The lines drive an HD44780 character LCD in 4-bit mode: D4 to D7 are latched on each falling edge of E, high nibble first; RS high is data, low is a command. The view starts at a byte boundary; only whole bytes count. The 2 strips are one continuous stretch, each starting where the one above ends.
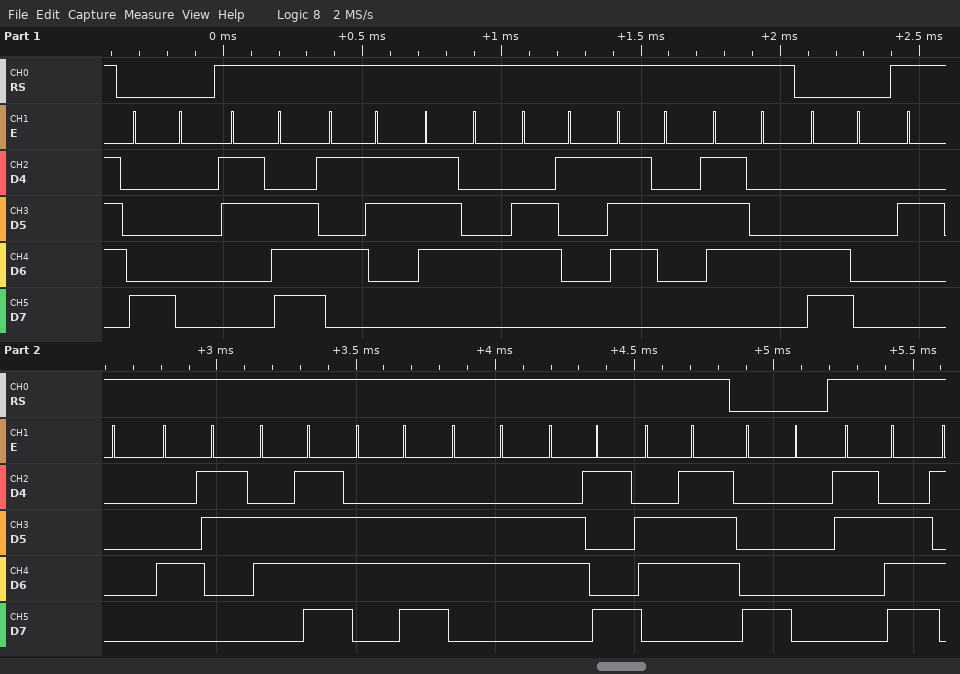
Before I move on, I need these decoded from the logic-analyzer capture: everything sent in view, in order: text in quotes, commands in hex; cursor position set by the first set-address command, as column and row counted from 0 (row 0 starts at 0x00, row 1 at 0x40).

0x80 ">Start" 0xC0 " Config" 0x80 ">"
column 0, row 0
